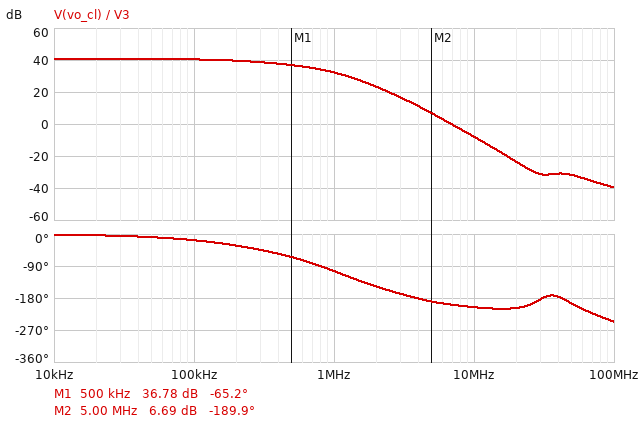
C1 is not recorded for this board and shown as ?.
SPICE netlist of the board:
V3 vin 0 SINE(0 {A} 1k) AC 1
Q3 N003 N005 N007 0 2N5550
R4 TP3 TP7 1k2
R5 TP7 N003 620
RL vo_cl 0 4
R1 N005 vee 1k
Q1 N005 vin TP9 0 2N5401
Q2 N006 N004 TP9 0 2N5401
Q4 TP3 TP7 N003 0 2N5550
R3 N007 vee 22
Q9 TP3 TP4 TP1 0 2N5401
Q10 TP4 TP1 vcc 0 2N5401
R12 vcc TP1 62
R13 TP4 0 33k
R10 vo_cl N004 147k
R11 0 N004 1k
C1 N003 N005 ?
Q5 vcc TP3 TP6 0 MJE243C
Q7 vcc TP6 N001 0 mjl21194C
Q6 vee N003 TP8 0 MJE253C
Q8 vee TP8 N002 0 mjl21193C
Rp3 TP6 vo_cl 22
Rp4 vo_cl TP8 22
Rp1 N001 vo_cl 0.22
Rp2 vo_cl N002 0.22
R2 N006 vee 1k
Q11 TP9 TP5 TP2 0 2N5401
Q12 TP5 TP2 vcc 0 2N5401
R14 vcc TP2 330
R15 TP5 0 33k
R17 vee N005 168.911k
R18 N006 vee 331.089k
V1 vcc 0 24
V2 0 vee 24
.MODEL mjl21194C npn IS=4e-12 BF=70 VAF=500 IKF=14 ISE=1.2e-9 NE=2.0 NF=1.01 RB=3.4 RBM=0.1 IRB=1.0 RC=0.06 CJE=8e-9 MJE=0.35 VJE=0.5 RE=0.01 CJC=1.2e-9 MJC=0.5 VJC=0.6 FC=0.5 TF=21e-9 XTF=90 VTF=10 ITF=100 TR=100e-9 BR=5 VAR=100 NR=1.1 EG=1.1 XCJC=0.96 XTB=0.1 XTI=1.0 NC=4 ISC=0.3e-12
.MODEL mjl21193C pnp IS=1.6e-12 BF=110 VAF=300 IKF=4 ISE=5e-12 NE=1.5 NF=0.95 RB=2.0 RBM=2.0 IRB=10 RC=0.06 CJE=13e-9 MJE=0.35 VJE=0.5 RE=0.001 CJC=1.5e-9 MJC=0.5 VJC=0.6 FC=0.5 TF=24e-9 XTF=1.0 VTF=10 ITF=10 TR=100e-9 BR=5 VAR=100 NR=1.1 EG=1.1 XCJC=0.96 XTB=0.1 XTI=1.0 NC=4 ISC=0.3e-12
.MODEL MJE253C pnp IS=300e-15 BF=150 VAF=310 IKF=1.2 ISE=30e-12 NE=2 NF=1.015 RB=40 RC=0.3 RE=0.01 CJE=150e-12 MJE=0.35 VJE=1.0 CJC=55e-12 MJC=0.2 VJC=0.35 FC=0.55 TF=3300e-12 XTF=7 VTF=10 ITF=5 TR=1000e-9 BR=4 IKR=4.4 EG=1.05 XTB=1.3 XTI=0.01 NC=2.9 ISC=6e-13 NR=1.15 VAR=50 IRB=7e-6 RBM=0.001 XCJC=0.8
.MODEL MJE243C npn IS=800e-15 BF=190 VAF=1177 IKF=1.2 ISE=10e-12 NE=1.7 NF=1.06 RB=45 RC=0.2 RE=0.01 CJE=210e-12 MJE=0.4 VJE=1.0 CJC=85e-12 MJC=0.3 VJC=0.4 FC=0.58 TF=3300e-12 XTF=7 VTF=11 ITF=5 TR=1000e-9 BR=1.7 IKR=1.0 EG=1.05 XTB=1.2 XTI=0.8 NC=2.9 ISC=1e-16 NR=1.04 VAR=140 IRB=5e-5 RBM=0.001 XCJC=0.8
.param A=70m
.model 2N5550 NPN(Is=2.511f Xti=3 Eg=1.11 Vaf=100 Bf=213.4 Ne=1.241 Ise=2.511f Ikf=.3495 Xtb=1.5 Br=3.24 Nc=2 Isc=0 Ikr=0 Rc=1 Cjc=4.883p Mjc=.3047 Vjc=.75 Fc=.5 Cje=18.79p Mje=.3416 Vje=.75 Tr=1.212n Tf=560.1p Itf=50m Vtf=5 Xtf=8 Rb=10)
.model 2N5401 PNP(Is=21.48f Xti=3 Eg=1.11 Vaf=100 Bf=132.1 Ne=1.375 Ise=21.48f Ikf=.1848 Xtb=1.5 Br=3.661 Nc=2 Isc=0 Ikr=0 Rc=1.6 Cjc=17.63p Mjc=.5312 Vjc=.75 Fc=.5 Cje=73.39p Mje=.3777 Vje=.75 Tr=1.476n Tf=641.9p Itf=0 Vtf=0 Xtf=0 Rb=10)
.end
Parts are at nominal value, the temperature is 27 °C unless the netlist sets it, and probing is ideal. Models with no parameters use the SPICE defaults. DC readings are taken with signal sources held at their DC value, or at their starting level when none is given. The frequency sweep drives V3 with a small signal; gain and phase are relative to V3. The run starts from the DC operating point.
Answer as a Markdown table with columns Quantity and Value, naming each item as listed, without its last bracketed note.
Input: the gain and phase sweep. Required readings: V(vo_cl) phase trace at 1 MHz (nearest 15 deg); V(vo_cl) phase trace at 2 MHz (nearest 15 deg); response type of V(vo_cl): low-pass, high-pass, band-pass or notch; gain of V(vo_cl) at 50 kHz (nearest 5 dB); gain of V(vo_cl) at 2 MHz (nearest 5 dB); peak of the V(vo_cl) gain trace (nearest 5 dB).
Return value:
| Quantity | Value |
|---|---|
| V(vo_cl) phase trace at 1 MHz | -105 deg |
| V(vo_cl) phase trace at 2 MHz | -150 deg |
| response type of V(vo_cl): low-pass, high-pass, band-pass or notch | low-pass |
| gain of V(vo_cl) at 50 kHz | 40 dB |
| gain of V(vo_cl) at 2 MHz | 25 dB |
| peak of the V(vo_cl) gain trace | 40 dB |
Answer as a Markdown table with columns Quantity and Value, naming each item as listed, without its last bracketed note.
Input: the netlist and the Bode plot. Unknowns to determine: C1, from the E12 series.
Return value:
| Quantity | Value |
|---|---|
| C1, from the E12 series | 10 pF |
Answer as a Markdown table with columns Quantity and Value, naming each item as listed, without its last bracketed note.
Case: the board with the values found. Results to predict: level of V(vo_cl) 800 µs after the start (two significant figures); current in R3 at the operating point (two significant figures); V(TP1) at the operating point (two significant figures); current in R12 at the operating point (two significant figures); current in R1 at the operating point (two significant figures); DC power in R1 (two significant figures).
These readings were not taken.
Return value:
| Quantity | Value |
|---|---|
| level of V(vo_cl) 800 µs after the start | -9.6 V |
| current in R3 at the operating point | 10 mA |
| V(TP1) at the operating point | 23 V |
| current in R12 at the operating point | 10 mA |
| current in R1 at the operating point | 970 µA |
| DC power in R1 | 940 µW |
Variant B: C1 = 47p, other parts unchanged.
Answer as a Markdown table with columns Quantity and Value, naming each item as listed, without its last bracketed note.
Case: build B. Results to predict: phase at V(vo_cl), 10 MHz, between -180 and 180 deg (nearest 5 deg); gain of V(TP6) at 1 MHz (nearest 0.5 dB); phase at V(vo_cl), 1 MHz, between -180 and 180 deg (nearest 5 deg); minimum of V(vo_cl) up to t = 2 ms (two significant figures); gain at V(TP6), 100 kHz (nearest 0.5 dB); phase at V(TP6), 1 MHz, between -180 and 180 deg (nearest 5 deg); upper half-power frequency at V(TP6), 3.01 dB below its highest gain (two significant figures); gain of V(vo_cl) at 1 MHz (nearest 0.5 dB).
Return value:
| Quantity | Value |
|---|---|
| phase at V(vo_cl), 10 MHz, between -180 and 180 deg | 150 deg |
| gain of V(TP6) at 1 MHz | 29.5 dB |
| phase at V(vo_cl), 1 MHz, between -180 and 180 deg | -110 deg |
| minimum of V(vo_cl) up to t = 2 ms | -10 V |
| gain at V(TP6), 100 kHz | 47.5 dB |
| phase at V(TP6), 1 MHz, between -180 and 180 deg | -130 deg |
| upper half-power frequency at V(TP6), 3.01 dB below its highest gain | 120 kHz |
| gain of V(vo_cl) at 1 MHz | 24.5 dB |
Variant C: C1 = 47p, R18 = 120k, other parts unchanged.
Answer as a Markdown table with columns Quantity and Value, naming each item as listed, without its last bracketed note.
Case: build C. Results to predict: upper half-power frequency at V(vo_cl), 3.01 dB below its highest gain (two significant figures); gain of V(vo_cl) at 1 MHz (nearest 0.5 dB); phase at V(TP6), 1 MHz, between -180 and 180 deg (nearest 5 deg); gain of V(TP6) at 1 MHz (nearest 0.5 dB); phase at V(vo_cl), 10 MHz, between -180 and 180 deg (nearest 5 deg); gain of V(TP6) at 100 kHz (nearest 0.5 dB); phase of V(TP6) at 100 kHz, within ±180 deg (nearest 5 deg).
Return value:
| Quantity | Value |
|---|---|
| upper half-power frequency at V(vo_cl), 3.01 dB below its highest gain | 120 kHz |
| gain of V(vo_cl) at 1 MHz | 24.5 dB |
| phase at V(TP6), 1 MHz, between -180 and 180 deg | -130 deg |
| gain of V(TP6) at 1 MHz | 29.5 dB |
| phase at V(vo_cl), 10 MHz, between -180 and 180 deg | 150 deg |
| gain of V(TP6) at 100 kHz | 47.5 dB |
| phase of V(TP6) at 100 kHz, within ±180 deg | -45 deg |
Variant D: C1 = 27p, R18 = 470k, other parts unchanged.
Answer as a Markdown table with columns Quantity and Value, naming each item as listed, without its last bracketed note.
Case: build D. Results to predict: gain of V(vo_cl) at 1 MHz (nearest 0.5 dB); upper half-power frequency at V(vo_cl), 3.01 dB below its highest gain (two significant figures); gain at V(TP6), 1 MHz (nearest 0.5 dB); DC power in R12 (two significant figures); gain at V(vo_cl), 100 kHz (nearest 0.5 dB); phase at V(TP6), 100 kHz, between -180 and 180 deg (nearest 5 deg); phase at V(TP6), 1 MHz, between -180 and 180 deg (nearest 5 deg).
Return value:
| Quantity | Value |
|---|---|
| gain of V(vo_cl) at 1 MHz | 28.0 dB |
| upper half-power frequency at V(vo_cl), 3.01 dB below its highest gain | 190 kHz |
| gain at V(TP6), 1 MHz | 33.0 dB |
| DC power in R12 | 6.3 mW |
| gain at V(vo_cl), 100 kHz | 39.5 dB |
| phase at V(TP6), 100 kHz, between -180 and 180 deg | -35 deg |
| phase at V(TP6), 1 MHz, between -180 and 180 deg | -130 deg |
